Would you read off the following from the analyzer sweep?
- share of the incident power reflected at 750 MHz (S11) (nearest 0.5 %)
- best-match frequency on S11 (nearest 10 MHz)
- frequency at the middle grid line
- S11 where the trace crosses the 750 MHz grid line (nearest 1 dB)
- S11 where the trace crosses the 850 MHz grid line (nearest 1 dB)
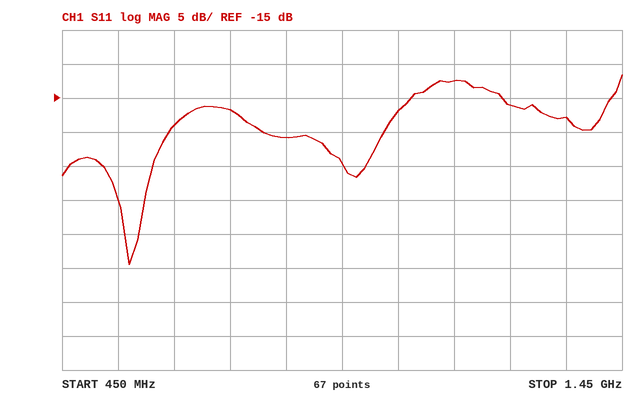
2.0 %
570 MHz
950 MHz
-17 dB
-21 dB
